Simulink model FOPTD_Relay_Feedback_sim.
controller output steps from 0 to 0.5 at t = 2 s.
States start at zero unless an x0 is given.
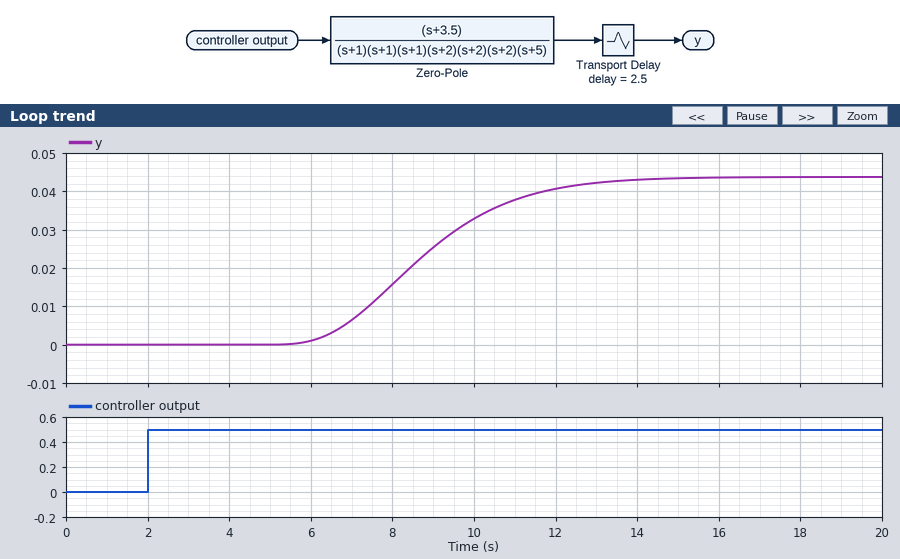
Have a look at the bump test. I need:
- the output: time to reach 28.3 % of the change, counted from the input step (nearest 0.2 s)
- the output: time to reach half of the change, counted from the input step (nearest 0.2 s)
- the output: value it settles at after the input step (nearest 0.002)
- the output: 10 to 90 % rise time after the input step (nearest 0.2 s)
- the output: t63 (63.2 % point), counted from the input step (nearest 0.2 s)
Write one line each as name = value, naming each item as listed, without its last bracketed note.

the output: time to reach 28.3 % of the change, counted from the input step = 5.6 s
the output: time to reach half of the change, counted from the input step = 6.6 s
the output: value it settles at after the input step = 0.044
the output: 10 to 90 % rise time after the input step = 4.8 s
the output: t63 (63.2 % point), counted from the input step = 7.2 s
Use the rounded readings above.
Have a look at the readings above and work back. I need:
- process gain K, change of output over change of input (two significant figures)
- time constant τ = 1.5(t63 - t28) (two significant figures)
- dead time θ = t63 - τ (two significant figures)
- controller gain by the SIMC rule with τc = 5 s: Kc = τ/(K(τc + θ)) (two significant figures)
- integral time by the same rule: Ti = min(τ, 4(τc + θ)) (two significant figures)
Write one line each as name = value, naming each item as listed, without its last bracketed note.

process gain K, change of output over change of input = 0.088
time constant τ = 1.5(t63 - t28) = 2.4 s
dead time θ = t63 - τ = 4.8 s
controller gain by the SIMC rule with τc = 5 s: Kc = τ/(K(τc + θ)) = 2.8
integral time by the same rule: Ti = min(τ, 4(τc + θ)) = 2.4 s
